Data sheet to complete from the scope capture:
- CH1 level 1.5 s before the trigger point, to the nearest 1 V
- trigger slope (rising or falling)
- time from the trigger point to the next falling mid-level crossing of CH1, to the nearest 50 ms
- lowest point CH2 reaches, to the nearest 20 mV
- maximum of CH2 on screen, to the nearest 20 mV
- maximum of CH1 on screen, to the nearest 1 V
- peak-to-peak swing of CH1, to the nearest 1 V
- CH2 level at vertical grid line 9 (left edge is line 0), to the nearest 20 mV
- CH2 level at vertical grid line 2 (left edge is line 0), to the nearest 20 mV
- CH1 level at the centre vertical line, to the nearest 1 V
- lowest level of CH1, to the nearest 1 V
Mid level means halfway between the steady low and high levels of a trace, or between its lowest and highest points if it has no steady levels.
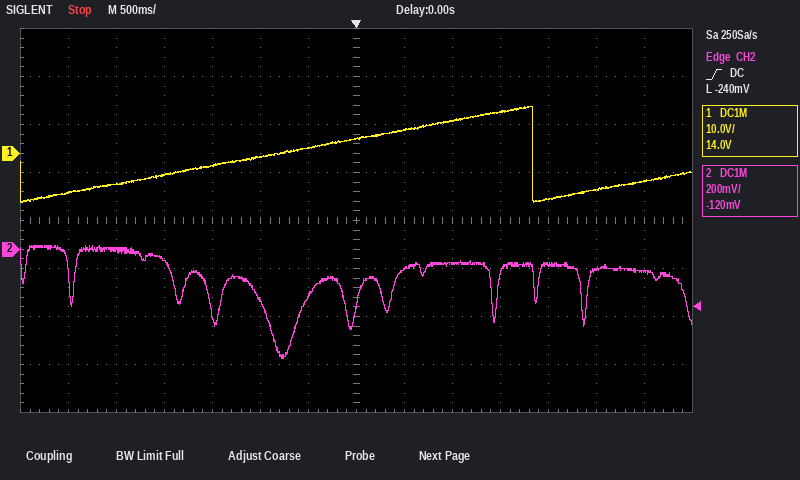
-3 V
rising
1.85 s
-460 mV
20 mV
10 V
20 V
-60 mV
0 mV
3 V
-10 V
